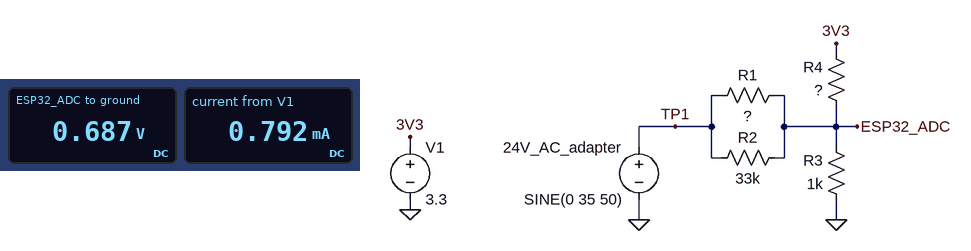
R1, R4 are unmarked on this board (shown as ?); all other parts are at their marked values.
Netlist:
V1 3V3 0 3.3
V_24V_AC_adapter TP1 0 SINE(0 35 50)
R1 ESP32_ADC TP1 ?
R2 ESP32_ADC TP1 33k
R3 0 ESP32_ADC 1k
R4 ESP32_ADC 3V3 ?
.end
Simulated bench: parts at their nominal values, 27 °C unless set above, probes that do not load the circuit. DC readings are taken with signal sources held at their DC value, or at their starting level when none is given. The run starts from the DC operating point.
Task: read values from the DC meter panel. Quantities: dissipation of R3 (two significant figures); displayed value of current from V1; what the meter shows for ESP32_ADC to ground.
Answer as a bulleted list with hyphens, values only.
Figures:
- 470 µW
- 0.792 mA
- 0.687 V
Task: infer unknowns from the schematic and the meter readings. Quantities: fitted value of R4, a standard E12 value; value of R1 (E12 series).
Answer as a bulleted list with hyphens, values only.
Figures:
- 3.3 kΩ
- 8.2 kΩ
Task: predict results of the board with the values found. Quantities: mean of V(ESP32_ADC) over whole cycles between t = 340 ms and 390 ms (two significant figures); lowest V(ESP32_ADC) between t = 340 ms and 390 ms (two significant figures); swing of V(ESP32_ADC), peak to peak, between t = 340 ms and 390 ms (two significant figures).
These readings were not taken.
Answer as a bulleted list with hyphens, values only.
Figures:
- 690 mV
- -3.0 V
- 7.3 V
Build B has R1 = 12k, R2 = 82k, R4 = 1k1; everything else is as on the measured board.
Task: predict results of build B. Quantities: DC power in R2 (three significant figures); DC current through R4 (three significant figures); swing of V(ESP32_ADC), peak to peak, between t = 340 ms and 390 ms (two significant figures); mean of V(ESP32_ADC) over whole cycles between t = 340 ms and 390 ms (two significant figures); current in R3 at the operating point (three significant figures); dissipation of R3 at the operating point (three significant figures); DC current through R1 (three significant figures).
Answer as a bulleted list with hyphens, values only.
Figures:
- 27.3 µW
- 1.64 mA
- 3.3 V
- 1.5 V
- 1.50 mA
- 2.24 mW
- 125 µA
